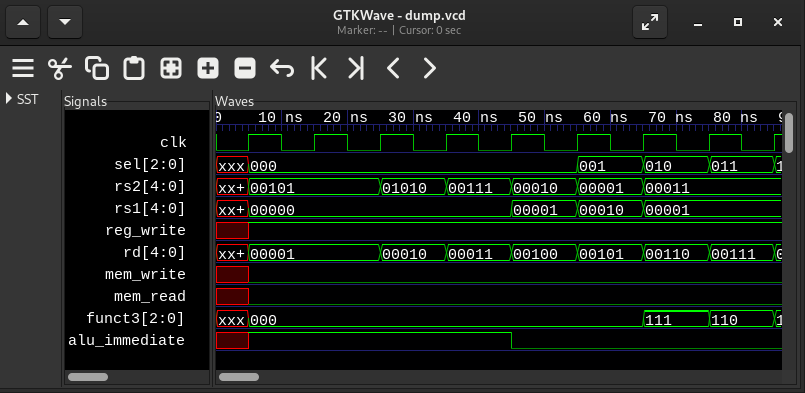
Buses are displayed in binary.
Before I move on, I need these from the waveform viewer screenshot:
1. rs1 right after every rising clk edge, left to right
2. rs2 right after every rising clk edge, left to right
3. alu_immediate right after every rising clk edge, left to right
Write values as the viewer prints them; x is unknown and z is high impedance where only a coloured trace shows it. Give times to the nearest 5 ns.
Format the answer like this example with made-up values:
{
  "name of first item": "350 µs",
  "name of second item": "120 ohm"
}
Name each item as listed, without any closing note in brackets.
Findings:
{
  "rs1 right after every rising clk edge, left to right": "00000, 00000, 00000, 00000, 00001, 00010, 00001, 00001, 00001",
  "rs2 right after every rising clk edge, left to right": "00101, 00101, 01010, 00111, 00010, 00001, 00011, 00011, 00011",
  "alu_immediate right after every rising clk edge, left to right": "1 1 1 1 0 0 0 0 0"
}
